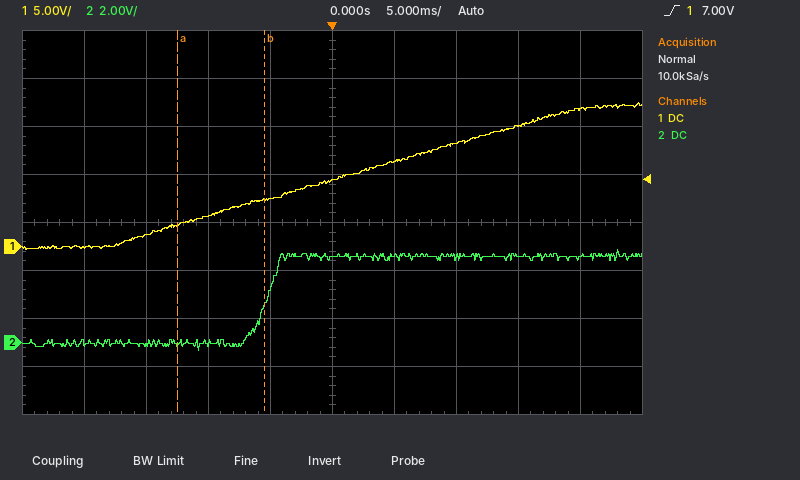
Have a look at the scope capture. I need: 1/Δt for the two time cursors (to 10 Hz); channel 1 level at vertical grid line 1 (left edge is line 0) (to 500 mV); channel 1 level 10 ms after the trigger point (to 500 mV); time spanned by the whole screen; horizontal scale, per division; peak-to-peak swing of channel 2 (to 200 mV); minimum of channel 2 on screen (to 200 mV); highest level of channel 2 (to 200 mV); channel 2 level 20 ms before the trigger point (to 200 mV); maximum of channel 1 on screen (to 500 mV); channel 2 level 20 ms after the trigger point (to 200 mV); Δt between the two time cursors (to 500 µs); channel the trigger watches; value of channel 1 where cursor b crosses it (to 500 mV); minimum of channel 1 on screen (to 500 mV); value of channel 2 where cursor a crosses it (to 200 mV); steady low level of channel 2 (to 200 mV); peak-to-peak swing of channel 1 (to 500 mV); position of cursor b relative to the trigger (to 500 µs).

140 Hz
0.0 V
11.0 V
50 ms
5 ms
4.2 V
-400 mV
3.8 V
0.0 V
15.0 V
3.6 V
7.0 ms
channel 1
5.0 V
-500 mV
0.0 V
0.0 V
15.5 V
-5.5 ms
